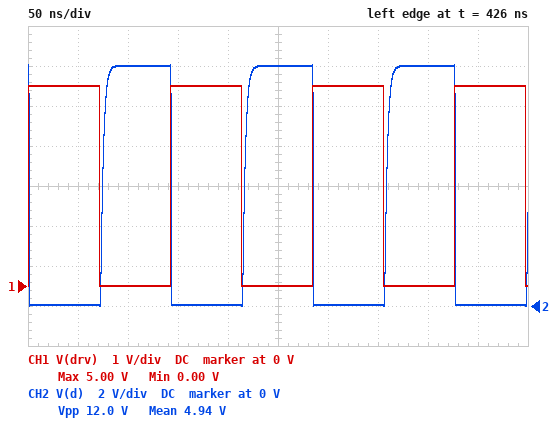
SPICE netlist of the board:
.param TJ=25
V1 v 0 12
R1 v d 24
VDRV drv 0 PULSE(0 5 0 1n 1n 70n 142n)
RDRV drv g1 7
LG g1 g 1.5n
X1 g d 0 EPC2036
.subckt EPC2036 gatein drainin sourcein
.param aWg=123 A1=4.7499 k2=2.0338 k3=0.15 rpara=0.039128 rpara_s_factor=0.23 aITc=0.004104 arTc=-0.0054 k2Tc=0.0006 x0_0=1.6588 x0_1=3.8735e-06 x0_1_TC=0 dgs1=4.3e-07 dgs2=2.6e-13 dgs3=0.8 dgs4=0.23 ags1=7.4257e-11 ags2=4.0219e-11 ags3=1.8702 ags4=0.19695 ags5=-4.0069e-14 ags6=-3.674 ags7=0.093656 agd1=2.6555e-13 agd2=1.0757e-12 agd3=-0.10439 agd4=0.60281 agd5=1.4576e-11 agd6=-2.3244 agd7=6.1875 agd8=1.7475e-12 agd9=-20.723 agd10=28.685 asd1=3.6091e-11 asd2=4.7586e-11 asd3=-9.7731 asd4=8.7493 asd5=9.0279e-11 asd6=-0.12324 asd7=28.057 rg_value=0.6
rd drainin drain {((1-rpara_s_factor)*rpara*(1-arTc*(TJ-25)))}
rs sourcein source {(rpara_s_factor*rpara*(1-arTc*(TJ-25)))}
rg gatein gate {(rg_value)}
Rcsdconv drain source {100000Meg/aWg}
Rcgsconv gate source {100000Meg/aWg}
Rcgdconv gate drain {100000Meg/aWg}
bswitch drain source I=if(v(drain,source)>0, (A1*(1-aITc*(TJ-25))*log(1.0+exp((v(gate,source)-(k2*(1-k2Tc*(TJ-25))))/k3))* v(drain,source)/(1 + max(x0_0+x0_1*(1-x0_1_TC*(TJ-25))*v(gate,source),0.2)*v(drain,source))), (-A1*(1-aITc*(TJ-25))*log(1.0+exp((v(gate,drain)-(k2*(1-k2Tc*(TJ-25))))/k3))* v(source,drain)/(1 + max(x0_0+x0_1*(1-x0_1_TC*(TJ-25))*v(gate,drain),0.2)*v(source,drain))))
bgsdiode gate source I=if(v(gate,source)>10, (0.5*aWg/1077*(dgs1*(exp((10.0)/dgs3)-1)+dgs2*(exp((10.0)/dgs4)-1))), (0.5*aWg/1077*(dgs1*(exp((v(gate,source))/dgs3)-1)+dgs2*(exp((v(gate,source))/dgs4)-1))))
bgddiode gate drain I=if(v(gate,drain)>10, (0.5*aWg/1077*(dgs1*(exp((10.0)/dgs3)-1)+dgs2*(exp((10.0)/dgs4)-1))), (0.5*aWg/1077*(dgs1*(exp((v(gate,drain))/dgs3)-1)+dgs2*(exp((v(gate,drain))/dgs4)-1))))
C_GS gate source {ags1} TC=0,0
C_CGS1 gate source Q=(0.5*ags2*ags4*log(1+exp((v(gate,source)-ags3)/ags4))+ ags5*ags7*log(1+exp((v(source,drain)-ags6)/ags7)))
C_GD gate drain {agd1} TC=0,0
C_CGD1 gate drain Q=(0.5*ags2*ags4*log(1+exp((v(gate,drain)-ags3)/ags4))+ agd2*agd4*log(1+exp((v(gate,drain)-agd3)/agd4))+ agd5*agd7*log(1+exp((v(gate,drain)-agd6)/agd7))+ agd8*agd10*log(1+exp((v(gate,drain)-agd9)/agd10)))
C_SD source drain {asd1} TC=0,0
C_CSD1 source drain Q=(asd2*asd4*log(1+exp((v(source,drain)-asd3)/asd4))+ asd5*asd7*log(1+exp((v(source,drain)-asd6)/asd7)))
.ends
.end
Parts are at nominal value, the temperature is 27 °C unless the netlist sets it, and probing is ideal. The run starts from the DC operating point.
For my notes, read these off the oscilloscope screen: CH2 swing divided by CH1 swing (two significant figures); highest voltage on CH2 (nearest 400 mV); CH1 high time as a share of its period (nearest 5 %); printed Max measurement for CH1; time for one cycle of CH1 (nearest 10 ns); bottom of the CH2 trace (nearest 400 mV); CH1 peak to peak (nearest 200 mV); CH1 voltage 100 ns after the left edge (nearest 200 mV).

2.4
12.0 V
50 %
5.00 V
140 ns
0 V
5.0 V
0 V
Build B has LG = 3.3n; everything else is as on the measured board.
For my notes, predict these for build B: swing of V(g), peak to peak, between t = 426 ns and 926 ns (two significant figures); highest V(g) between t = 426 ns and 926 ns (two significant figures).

5.4 V
5.2 V
